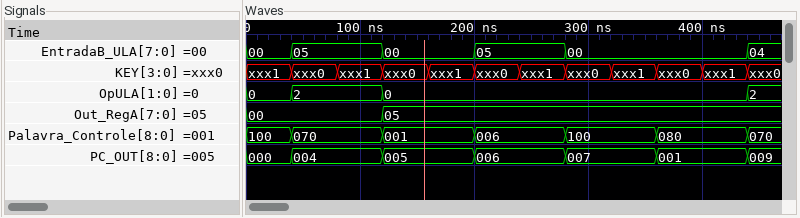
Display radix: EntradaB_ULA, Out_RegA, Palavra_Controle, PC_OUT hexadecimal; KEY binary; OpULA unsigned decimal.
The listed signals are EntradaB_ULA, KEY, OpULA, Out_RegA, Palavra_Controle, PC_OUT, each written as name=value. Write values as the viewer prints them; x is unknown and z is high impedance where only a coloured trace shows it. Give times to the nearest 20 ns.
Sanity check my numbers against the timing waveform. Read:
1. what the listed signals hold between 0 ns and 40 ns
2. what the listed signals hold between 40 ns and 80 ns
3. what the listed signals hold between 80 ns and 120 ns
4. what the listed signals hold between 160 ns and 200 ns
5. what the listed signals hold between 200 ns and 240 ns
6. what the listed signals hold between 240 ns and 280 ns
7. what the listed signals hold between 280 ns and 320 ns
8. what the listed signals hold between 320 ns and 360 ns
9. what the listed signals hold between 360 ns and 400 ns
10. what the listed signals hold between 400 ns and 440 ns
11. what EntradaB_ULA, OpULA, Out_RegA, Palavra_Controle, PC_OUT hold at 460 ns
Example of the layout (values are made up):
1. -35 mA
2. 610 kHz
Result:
1. EntradaB_ULA=00, KEY=xxx1, OpULA=0, Out_RegA=00, Palavra_Controle=100, PC_OUT=000
2. EntradaB_ULA=05, KEY=xxx0, OpULA=2, Out_RegA=00, Palavra_Controle=070, PC_OUT=004
3. EntradaB_ULA=05, KEY=xxx1, OpULA=2, Out_RegA=00, Palavra_Controle=070, PC_OUT=004
4. EntradaB_ULA=00, KEY=xxx1, OpULA=0, Out_RegA=05, Palavra_Controle=001, PC_OUT=005
5. EntradaB_ULA=05, KEY=xxx0, OpULA=0, Out_RegA=05, Palavra_Controle=006, PC_OUT=006
6. EntradaB_ULA=05, KEY=xxx1, OpULA=0, Out_RegA=05, Palavra_Controle=006, PC_OUT=006
7. EntradaB_ULA=00, KEY=xxx0, OpULA=0, Out_RegA=05, Palavra_Controle=100, PC_OUT=007
8. EntradaB_ULA=00, KEY=xxx1, OpULA=0, Out_RegA=05, Palavra_Controle=100, PC_OUT=007
9. EntradaB_ULA=00, KEY=xxx0, OpULA=0, Out_RegA=05, Palavra_Controle=080, PC_OUT=001
10. EntradaB_ULA=00, KEY=xxx1, OpULA=0, Out_RegA=05, Palavra_Controle=080, PC_OUT=001
11. EntradaB_ULA=04, OpULA=2, Out_RegA=05, Palavra_Controle=070, PC_OUT=009
